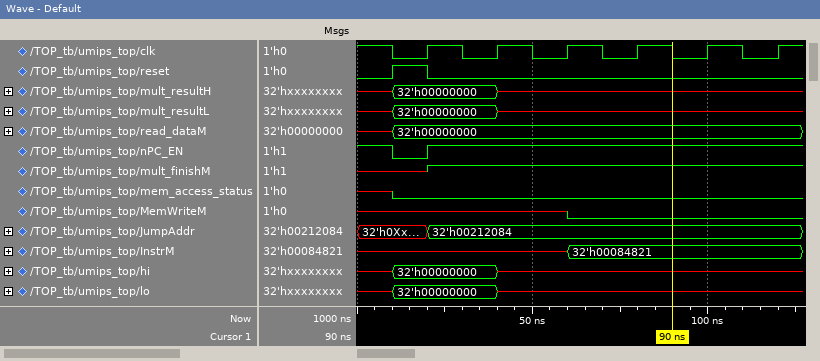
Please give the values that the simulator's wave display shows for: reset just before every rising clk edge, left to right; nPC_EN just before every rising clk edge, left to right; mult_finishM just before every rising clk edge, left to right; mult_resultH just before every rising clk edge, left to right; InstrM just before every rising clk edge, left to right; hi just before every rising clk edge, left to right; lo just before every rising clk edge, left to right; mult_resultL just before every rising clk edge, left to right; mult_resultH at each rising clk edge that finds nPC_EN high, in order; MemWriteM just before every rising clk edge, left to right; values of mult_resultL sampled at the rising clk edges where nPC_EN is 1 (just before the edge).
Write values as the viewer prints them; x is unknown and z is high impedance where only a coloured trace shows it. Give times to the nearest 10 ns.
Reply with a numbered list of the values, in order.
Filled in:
1. 1 0 0 0 0 0
2. 0 1 1 1 1 1
3. x 1 1 1 1 1
4. 32'h00000000, 32'h00000000, x, x, x, x
5. x, x, x, 32'h00084821, 32'h00084821, 32'h00084821
6. 32'h00000000, 32'h00000000, x, x, x, x
7. 32'h00000000, 32'h00000000, x, x, x, x
8. 32'h00000000, 32'h00000000, x, x, x, x
9. 32'h00000000, x, x, x, x
10. x x x 0 0 0
11. 32'h00000000, x, x, x, x
